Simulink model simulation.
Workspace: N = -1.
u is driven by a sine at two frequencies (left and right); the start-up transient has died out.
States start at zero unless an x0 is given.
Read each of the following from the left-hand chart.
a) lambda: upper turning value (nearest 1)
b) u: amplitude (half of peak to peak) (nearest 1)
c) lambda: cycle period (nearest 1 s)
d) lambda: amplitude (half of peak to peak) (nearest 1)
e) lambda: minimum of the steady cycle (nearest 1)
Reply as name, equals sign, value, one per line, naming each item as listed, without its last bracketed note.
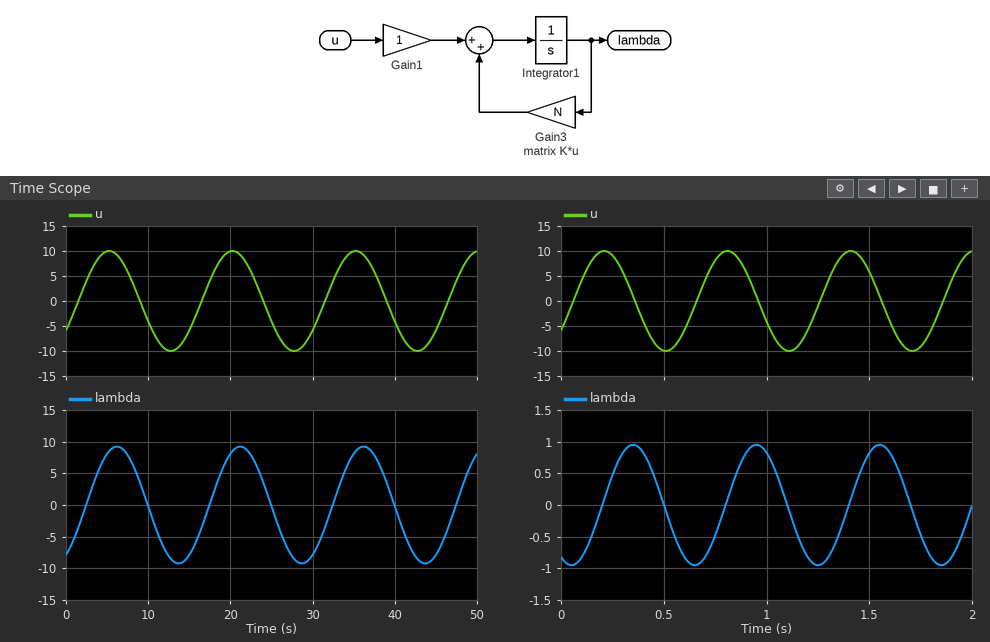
lambda: upper turning value = 9
u: amplitude (half of peak to peak) = 10
lambda: cycle period = 15 s
lambda: amplitude (half of peak to peak) = 9
lambda: minimum of the steady cycle = -9
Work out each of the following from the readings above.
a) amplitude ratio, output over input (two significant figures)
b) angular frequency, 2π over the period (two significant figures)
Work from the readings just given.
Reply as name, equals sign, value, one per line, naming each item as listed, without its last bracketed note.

amplitude ratio, output over input = 0.90
angular frequency, 2π over the period = 0.42 rad/s
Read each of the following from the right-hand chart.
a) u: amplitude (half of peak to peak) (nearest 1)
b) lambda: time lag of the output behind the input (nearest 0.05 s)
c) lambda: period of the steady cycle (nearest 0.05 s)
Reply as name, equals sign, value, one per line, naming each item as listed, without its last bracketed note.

u: amplitude (half of peak to peak) = 10
lambda: time lag of the output behind the input = 0.15 s
lambda: period of the steady cycle = 0.60 s
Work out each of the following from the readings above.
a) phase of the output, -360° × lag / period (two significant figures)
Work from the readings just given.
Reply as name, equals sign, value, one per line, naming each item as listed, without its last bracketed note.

phase of the output, -360° × lag / period = -90°
